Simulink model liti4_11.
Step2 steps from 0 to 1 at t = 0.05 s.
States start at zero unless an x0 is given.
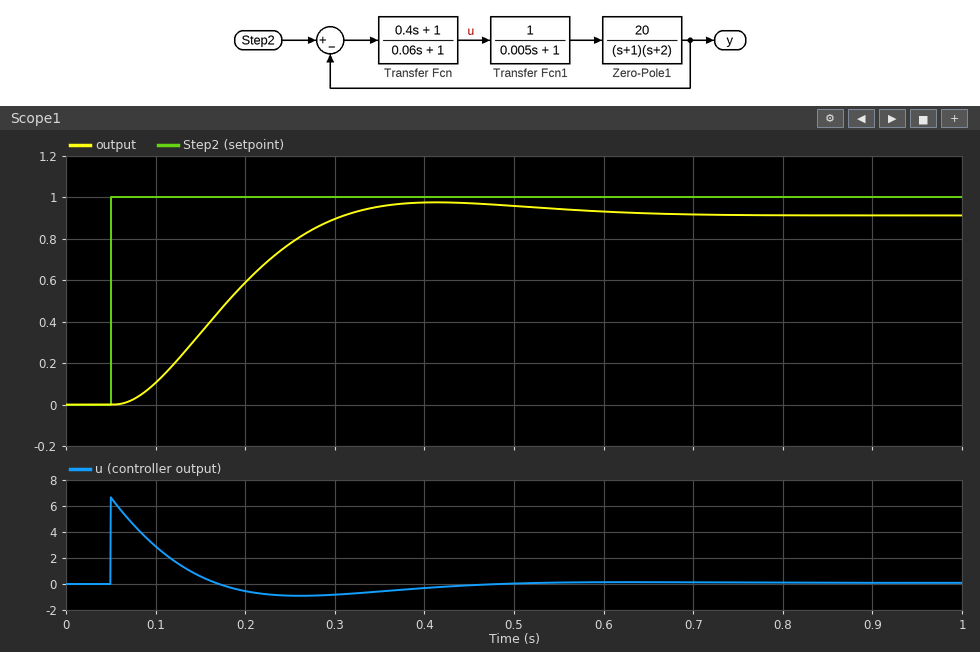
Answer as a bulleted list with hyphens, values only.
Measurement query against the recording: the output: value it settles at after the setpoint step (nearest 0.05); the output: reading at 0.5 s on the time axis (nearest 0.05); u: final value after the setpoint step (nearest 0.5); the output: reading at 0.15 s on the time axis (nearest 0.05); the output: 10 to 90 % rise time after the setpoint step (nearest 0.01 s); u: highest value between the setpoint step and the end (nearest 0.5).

- 0.90
- 0.95
- 0.0
- 0.35
- 0.17 s
- 6.5
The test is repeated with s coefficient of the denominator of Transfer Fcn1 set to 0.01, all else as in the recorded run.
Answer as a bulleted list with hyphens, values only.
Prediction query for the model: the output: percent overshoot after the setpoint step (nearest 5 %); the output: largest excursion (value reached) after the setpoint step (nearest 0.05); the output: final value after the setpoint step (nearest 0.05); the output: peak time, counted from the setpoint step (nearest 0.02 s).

- 10 %
- 1.00
- 0.90
- 0.36 s
